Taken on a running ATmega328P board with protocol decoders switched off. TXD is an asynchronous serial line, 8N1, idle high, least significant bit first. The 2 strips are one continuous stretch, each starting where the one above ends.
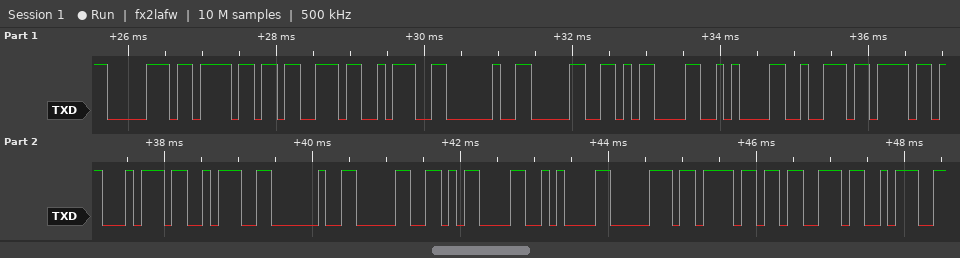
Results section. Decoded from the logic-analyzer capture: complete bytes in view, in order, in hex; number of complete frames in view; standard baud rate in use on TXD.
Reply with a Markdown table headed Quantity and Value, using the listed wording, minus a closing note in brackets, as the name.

| Quantity | Value |
|---|---|
| complete bytes in view, in order, in hex | 70 6F 73 3A 20 30 0D 0A 72 6F 74 3A 20 30 0D 0A 70 6F 73 3A |
| number of complete frames in view | 20 |
| standard baud rate in use on TXD | 9600 baud |
